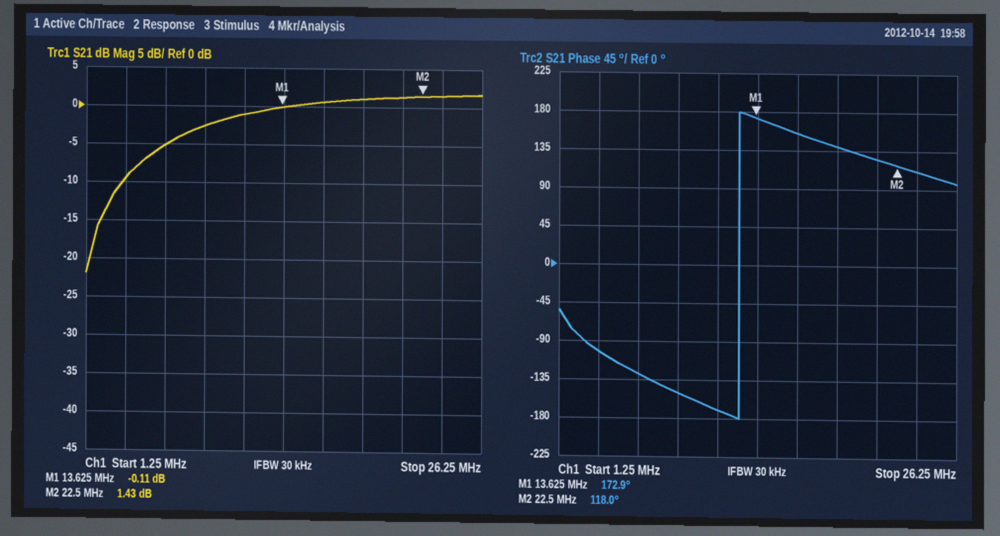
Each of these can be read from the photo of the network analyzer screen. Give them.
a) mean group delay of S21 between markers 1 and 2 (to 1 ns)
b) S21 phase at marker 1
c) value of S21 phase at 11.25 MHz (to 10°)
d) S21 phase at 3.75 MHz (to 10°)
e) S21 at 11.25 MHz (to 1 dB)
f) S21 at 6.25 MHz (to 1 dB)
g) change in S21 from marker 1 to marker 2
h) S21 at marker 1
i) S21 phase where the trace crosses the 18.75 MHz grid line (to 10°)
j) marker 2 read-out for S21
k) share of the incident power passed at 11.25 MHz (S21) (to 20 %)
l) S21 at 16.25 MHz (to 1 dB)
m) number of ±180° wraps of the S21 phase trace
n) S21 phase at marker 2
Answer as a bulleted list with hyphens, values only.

- 17 ns
- 172.9°
- -170°
- -100°
- -1 dB
- -5 dB
- 1.54 dB
- -0.11 dB
- 140°
- 1.43 dB
- 80 %
- 1 dB
- 1
- 118.0°
